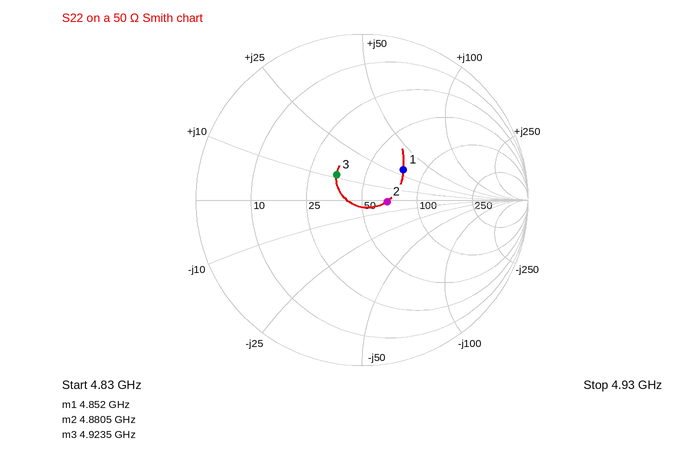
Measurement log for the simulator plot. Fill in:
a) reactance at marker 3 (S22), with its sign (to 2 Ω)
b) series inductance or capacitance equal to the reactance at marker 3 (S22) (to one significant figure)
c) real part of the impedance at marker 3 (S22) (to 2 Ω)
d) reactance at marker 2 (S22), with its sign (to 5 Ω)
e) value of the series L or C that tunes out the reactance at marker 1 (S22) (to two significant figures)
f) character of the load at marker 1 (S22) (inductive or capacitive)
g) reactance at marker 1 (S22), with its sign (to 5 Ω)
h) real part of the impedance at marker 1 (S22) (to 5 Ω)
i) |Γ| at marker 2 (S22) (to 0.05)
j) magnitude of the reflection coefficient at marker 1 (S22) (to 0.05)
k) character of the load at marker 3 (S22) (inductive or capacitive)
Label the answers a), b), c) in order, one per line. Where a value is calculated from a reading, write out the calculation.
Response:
a) +12 Ω
b) L = 12 Ω/(2π × 4.9235 GHz) ≈ 388 pH, so 400 pH to one significant figure
c) 36 Ω
d) 0 Ω
e) C = 1/(2π × 4.852 GHz × 30 Ω) ≈ 1.1 pF
f) inductive
g) +30 Ω
h) 75 Ω
i) 0.15
j) 0.30
k) inductive
